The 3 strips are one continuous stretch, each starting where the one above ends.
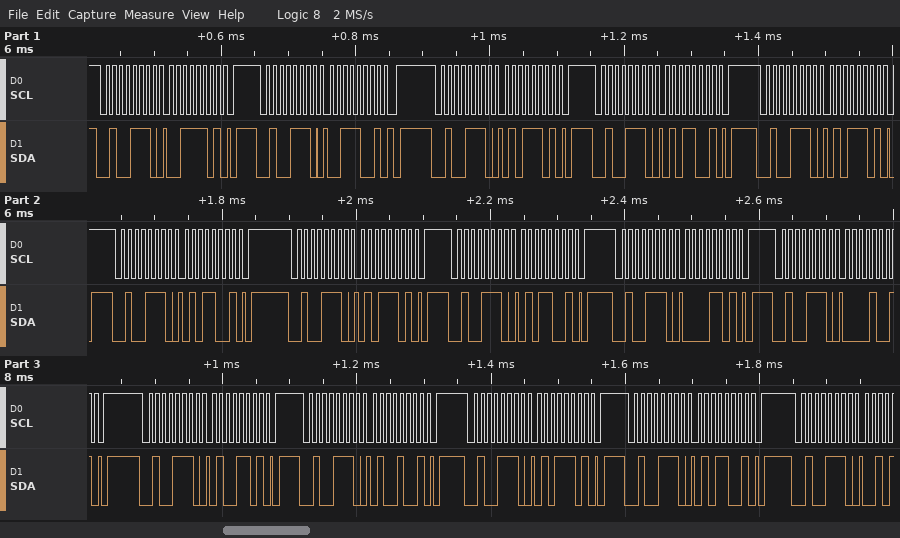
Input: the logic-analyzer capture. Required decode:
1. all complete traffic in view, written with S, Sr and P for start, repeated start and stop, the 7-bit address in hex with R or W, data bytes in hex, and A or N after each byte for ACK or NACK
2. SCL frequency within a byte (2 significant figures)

S 27W A 3D A P S 27W A 39 A P S 27W A 5D A P S 27W A 59 A P S 27W A 5D A P S 27W A 59 A P S 27W A 5D A P S 27W A 59 A P S 27W A 0D A P S 27W A 09 A P S 27W A 4D A P S 27W A 49 A P S 27W A 5D A P S 27W A 59 A P S 27W A
100 kHz
